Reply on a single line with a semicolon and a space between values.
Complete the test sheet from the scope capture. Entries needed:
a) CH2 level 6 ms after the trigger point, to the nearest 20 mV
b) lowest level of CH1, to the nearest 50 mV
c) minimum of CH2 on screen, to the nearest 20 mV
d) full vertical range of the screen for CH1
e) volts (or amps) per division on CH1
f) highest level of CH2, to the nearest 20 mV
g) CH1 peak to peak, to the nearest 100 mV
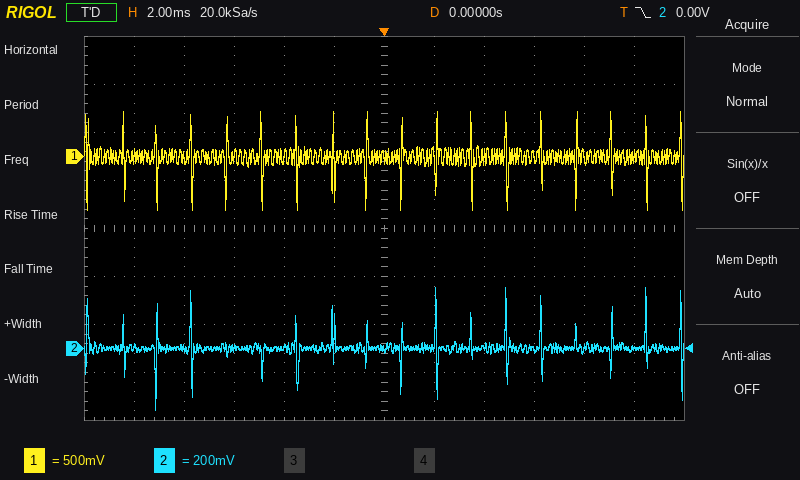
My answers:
0 mV; -550 mV; -260 mV; 4 V; 500 mV; 260 mV; 1.00 V
